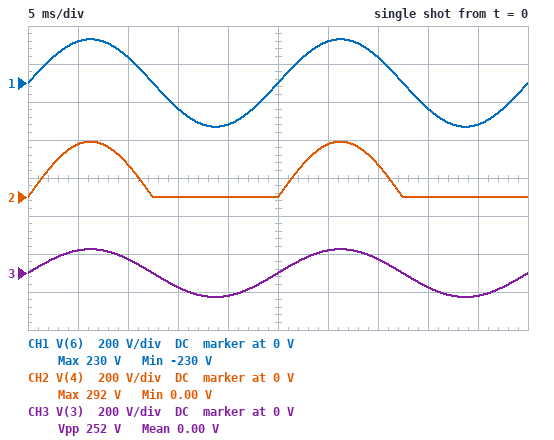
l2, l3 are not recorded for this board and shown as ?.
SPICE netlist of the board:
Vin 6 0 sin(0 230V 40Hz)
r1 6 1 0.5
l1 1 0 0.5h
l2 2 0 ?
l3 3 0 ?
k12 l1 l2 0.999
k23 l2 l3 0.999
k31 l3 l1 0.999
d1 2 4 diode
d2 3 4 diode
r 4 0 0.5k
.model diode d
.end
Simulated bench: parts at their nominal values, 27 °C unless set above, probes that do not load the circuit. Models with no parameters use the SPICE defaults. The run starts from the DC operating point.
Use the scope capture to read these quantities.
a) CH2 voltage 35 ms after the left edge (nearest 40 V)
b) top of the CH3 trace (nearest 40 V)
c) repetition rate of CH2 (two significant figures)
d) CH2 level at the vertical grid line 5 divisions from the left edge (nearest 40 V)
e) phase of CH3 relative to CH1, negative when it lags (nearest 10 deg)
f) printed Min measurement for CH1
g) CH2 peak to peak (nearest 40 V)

160 V
120 V
40 Hz
0 V
0 deg
-230 V
280 V
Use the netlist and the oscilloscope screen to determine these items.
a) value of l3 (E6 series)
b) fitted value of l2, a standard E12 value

150 mH
820 mH
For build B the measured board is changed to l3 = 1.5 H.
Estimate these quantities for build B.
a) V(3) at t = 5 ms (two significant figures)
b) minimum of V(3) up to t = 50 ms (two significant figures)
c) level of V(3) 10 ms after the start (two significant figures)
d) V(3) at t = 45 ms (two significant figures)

380 V
-400 V
230 V
-380 V
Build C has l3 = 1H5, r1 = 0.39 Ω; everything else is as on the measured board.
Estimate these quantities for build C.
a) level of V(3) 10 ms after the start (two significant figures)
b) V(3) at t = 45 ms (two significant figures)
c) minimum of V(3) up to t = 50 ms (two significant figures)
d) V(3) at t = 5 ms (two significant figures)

230 V
-380 V
-400 V
380 V
